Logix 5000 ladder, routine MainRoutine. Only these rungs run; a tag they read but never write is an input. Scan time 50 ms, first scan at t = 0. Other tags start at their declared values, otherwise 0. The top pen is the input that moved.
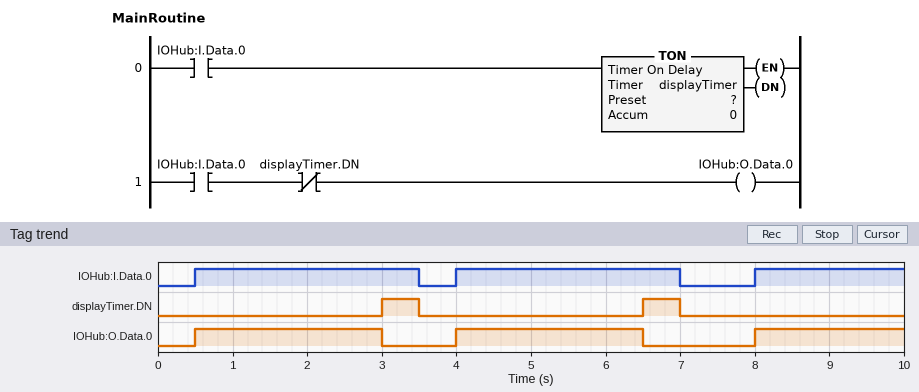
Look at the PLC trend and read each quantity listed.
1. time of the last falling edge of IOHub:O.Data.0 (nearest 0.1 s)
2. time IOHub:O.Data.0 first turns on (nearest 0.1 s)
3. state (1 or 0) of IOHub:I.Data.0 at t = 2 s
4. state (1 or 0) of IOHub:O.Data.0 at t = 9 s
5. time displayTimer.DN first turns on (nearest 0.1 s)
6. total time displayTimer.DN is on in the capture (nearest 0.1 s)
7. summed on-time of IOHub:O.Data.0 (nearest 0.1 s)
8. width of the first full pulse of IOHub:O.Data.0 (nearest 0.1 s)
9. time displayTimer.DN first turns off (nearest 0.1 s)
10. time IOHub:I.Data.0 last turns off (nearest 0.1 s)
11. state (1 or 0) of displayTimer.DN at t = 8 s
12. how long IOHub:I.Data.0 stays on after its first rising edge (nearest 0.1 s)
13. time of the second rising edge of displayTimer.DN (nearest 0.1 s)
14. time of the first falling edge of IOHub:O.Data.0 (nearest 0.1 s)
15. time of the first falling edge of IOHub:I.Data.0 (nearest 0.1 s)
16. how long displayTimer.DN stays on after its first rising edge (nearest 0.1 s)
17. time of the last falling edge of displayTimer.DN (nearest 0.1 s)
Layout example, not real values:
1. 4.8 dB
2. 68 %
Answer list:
1. 6.5 s
2. 0.5 s
3. 1
4. 1
5. 3.0 s
6. 1.0 s
7. 7.0 s
8. 2.5 s
9. 3.5 s
10. 7.0 s
11. 0
12. 3.0 s
13. 6.5 s
14. 3.0 s
15. 3.5 s
16. 0.5 s
17. 7.0 s
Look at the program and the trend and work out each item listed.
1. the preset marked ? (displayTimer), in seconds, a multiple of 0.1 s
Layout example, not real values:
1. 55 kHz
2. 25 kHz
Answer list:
1. 2.5 s
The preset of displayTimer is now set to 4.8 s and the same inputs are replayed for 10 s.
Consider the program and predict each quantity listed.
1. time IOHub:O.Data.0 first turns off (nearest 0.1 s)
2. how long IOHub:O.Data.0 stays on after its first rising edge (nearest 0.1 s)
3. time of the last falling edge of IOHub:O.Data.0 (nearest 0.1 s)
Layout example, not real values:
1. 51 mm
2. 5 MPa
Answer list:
1. 3.5 s
2. 3.0 s
3. 7.0 s
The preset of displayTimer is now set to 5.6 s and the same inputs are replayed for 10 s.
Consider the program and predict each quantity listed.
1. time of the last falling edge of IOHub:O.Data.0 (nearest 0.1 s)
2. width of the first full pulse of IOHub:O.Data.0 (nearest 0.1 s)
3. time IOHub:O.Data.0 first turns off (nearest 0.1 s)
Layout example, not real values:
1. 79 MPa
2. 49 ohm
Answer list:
1. 7.0 s
2. 3.0 s
3. 3.5 s
